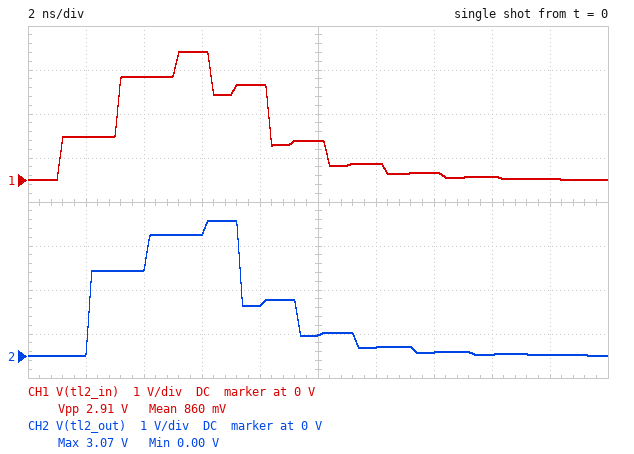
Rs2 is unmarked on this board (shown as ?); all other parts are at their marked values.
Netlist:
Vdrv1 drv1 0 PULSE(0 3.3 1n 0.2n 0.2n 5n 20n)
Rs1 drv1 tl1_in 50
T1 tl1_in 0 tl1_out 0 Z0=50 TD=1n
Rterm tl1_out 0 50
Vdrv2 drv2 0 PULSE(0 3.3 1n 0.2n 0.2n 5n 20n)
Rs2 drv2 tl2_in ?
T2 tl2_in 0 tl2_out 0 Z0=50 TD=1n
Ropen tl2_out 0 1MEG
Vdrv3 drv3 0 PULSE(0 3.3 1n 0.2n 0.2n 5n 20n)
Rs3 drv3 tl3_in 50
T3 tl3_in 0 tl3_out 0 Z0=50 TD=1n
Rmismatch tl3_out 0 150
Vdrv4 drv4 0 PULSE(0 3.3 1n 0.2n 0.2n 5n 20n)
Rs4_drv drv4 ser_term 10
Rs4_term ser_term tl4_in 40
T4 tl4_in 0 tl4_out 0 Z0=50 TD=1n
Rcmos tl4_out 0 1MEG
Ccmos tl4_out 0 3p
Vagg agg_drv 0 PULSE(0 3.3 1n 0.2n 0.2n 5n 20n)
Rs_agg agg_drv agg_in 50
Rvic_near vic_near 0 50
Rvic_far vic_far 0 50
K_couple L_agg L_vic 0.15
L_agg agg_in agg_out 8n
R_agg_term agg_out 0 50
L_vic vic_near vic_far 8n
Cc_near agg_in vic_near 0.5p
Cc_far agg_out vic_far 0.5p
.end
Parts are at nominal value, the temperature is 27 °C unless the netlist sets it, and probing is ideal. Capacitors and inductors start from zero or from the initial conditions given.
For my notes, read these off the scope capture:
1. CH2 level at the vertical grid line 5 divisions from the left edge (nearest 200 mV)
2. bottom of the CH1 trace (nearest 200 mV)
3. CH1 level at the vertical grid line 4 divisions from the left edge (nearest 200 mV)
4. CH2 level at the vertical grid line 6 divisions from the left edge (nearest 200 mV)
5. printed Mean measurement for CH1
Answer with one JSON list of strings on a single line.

["400 mV", "0 V", "2.2 V", "200 mV", "860 mV"]
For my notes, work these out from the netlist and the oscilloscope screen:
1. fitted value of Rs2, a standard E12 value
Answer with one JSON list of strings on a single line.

["120 Ω"]
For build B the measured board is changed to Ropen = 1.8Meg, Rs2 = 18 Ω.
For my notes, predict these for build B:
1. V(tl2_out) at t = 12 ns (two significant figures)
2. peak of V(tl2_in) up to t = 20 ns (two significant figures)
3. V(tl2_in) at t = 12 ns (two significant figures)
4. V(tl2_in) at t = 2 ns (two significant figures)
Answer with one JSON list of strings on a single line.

["-270 mV", "3.7 V", "210 mV", "2.4 V"]
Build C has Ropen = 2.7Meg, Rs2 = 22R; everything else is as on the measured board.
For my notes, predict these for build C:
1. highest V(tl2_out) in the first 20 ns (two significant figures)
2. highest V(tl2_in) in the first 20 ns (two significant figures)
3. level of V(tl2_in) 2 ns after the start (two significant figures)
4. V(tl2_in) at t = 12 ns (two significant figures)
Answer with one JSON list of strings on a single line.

["4.6 V", "3.7 V", "2.3 V", "160 mV"]
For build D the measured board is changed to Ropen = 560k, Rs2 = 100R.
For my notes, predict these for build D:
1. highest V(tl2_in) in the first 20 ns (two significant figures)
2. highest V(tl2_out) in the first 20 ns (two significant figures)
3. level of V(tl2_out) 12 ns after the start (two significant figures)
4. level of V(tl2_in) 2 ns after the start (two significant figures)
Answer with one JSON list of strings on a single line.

["3.1 V", "3.2 V", "110 mV", "1.1 V"]
